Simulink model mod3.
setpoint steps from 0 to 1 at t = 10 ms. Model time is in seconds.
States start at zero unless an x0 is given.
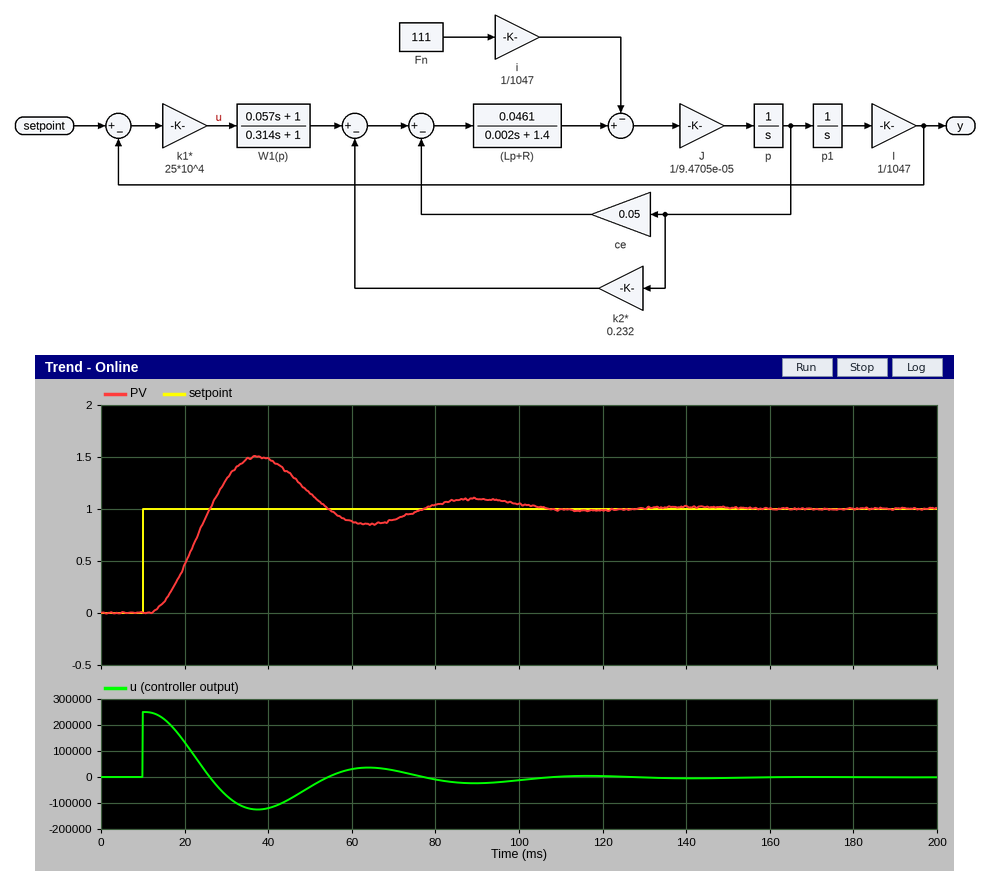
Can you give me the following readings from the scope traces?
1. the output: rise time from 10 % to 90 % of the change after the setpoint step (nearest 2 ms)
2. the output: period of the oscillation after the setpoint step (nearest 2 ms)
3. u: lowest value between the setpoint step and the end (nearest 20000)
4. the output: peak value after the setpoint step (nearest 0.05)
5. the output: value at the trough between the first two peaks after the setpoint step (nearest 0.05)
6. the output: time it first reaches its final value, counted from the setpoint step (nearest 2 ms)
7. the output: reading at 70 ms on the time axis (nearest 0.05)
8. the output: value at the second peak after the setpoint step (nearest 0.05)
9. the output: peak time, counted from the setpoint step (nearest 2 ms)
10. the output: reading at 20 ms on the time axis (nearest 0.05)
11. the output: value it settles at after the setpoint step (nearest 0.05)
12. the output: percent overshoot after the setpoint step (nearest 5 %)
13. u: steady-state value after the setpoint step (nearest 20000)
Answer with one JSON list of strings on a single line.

["10 ms", "52 ms", "-120000", "1.50", "0.85", "16 ms", "0.90", "1.10", "28 ms", "0.45", "1.00", "50 %", "0"]
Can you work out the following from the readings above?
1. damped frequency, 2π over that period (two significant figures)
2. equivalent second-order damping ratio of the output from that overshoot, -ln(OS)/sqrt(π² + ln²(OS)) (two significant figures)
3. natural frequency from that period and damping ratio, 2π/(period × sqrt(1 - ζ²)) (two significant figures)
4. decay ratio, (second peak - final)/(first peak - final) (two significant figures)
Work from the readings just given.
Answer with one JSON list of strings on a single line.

["0.12 rad/ms", "0.22", "0.12 rad/ms", "0.20"]
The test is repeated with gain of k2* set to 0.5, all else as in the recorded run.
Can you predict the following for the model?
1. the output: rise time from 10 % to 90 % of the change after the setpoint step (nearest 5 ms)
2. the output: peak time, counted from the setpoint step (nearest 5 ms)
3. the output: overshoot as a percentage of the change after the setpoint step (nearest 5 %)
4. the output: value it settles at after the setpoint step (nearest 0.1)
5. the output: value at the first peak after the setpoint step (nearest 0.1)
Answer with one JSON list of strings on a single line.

["15 ms", "35 ms", "15 %", "1.0", "1.2"]
